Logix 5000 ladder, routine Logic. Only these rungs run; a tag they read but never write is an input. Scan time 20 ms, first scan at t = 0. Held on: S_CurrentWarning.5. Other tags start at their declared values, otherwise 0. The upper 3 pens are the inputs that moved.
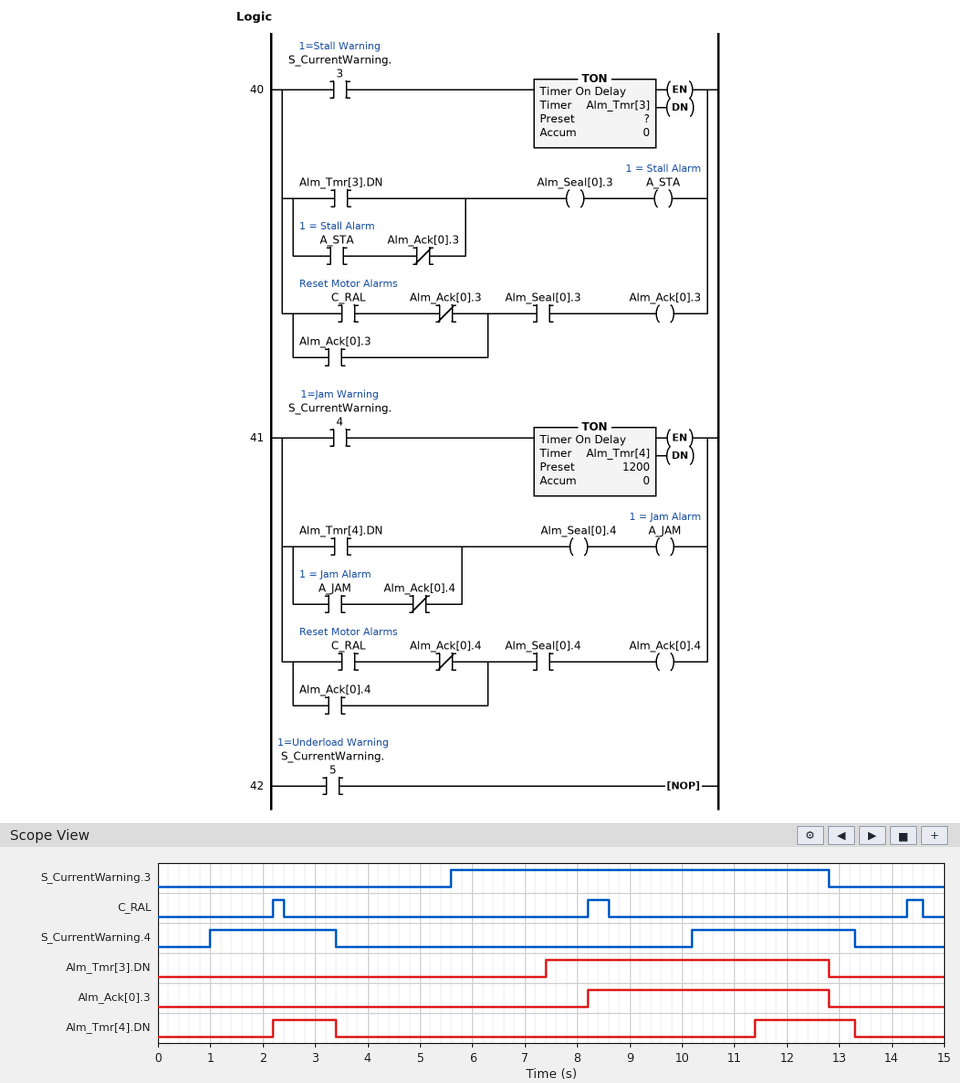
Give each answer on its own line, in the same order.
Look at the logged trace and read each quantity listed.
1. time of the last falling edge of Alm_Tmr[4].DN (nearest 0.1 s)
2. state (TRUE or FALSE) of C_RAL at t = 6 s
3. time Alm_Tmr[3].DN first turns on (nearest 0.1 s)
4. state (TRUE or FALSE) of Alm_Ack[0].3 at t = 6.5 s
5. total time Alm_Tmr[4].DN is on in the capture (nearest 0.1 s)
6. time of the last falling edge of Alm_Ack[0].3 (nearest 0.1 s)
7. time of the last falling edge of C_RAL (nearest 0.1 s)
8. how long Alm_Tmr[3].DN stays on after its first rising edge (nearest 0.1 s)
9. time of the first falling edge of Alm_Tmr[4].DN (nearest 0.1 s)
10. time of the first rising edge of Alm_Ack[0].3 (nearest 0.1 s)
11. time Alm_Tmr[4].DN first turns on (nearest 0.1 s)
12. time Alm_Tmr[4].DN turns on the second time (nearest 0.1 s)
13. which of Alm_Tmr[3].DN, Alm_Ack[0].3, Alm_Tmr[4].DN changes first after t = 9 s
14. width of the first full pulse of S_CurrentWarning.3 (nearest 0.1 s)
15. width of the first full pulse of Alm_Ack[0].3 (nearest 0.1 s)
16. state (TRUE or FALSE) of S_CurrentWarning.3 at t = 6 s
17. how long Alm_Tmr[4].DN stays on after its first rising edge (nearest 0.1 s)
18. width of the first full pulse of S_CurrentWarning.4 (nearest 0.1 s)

13.3 s
FALSE
7.4 s
FALSE
3.1 s
12.8 s
14.6 s
5.4 s
3.4 s
8.2 s
2.2 s
11.4 s
Alm_Tmr[4].DN
7.2 s
4.6 s
TRUE
1.2 s
2.4 s
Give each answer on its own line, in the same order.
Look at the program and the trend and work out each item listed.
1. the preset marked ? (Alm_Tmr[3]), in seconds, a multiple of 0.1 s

1.8 s
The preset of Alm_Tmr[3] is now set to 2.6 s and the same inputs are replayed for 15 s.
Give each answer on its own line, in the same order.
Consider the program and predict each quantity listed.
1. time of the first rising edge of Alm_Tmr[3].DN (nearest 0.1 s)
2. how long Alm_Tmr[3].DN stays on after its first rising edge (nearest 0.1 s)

8.2 s
4.6 s
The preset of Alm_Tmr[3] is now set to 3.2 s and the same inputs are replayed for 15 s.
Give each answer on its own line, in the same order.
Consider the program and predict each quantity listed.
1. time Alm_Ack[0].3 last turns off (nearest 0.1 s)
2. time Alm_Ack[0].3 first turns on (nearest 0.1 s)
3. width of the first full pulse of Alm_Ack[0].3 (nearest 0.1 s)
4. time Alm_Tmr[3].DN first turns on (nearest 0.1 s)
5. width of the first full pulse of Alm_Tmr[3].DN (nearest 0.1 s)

14.3 s
14.3 s
0.0 s
8.8 s
4.0 s
